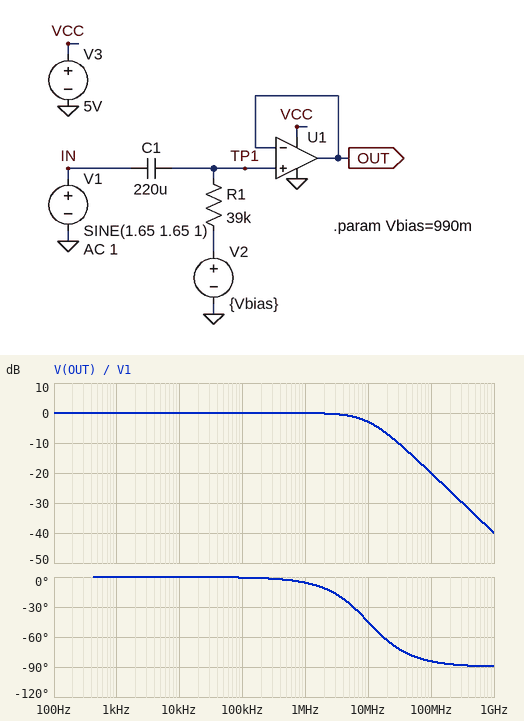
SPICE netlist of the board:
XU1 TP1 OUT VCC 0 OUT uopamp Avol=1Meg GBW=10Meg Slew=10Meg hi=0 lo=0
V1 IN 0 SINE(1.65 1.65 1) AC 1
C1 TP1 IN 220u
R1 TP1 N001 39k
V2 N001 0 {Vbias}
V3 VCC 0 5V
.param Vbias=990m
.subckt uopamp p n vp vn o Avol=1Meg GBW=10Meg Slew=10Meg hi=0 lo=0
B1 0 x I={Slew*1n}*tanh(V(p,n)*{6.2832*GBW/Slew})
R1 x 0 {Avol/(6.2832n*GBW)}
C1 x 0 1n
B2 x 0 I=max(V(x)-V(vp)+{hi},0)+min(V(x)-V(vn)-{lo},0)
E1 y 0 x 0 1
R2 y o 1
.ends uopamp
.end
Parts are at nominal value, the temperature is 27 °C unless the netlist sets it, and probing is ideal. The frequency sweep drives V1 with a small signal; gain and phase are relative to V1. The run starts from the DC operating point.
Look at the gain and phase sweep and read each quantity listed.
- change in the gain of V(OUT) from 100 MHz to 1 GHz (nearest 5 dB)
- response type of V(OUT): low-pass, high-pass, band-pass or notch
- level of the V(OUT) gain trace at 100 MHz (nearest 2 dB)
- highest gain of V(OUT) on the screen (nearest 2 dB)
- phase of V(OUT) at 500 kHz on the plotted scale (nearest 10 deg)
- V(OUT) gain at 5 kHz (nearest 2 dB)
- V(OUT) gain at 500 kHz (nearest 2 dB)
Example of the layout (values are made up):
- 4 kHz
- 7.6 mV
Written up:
- -20 dB
- low-pass
- -20 dB
- 0 dB
- 0 deg
- 0 dB
- 0 dB
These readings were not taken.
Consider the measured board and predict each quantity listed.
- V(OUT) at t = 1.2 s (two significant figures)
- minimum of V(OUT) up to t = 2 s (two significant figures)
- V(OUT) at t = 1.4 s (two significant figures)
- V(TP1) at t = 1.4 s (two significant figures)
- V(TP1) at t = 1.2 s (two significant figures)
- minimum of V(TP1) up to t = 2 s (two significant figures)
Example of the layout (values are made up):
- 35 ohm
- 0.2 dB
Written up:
- 2.5 V
- -10 mV
- 1.9 V
- 1.9 V
- 2.5 V
- -690 mV
